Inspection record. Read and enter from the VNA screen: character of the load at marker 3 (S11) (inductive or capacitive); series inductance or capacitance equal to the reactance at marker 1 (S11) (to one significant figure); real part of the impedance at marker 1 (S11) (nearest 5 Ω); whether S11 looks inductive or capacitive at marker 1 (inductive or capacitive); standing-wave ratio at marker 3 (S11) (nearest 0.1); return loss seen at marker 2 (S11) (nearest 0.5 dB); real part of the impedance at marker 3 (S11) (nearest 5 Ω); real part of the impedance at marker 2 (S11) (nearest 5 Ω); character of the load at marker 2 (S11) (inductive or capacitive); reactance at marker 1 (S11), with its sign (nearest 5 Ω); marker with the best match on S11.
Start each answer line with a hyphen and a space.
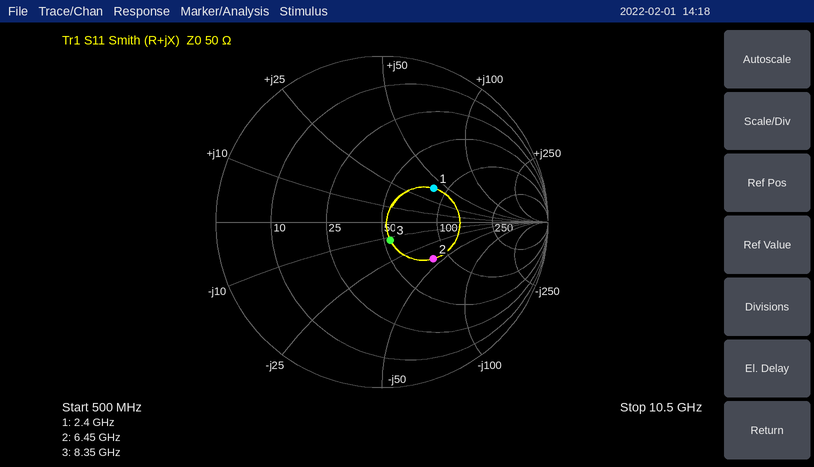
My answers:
- capacitive
- 3 nH
- 85 Ω
- inductive
- 1.3
- 8.5 dB
- 55 Ω
- 80 Ω
- capacitive
- +40 Ω
- marker 3
